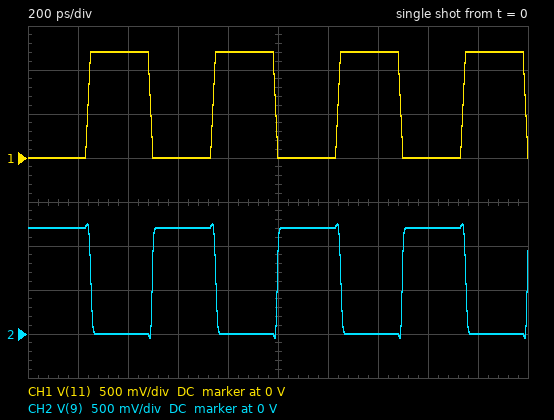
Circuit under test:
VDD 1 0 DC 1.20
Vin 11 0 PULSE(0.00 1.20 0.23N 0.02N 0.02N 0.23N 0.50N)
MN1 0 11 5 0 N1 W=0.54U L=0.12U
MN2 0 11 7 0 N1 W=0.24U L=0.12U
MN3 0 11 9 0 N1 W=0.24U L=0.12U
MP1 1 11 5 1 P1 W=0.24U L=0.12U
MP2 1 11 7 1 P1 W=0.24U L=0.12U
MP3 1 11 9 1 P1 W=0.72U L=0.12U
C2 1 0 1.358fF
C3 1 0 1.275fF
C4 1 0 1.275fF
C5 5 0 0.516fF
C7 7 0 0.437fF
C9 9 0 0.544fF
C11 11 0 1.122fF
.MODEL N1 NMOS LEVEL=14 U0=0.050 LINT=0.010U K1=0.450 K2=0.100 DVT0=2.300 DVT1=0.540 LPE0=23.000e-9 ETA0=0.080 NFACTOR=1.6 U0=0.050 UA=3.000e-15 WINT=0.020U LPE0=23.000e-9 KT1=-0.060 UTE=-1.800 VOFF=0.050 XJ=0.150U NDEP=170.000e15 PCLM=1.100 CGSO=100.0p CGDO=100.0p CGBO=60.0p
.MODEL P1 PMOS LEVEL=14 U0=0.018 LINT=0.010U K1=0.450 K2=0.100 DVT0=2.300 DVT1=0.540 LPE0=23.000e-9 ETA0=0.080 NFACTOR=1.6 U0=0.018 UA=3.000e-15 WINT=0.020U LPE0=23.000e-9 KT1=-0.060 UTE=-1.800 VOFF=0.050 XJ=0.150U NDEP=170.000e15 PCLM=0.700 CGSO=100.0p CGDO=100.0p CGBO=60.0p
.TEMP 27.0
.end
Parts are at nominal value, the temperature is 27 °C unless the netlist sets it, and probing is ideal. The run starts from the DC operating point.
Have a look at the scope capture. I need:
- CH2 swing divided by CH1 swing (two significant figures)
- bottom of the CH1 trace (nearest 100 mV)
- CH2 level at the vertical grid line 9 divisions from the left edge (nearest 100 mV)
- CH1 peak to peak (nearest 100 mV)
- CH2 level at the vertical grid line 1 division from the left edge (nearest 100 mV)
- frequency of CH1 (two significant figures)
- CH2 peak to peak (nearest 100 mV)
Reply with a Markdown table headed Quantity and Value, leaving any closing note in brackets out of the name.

| Quantity | Value |
|---|---|
| CH2 swing divided by CH1 swing | 1.1 |
| bottom of the CH1 trace | 0 V |
| CH2 level at the vertical grid line 9 divisions from the left edge | 0 V |
| CH1 peak to peak | 1.2 V |
| CH2 level at the vertical grid line 1 division from the left edge | 1.2 V |
| frequency of CH1 | 2.0 GHz |
| CH2 peak to peak | 1.3 V |
